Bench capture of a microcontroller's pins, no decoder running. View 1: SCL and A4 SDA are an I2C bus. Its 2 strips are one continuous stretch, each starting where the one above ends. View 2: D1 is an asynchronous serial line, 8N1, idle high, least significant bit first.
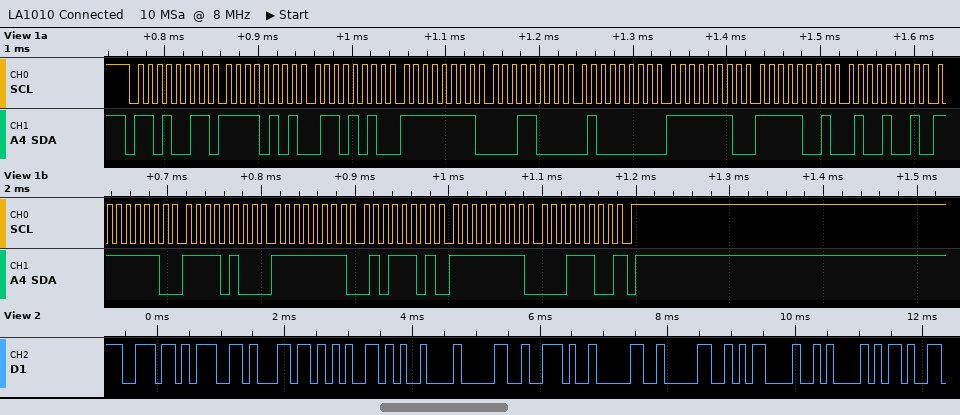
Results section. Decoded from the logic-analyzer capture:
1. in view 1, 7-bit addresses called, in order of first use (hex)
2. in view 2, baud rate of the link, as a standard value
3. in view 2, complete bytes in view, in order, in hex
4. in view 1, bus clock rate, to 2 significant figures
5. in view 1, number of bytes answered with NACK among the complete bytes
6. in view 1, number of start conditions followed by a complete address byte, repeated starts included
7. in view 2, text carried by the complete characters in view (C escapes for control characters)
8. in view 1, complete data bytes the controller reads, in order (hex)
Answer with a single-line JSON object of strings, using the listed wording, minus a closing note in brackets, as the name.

{"in view 1, 7-bit addresses called, in order of first use": "0x69", "in view 2, baud rate of the link, as a standard value": "9600 baud", "in view 2, complete bytes in view, in order, in hex": "6E 67 6C 65 09 30 2E 30 30 0D 0A 2D", "in view 1, bus clock rate, to 2 significant figures": "100 kHz", "in view 1, number of bytes answered with NACK among the complete bytes": "1", "in view 1, number of start conditions followed by a complete address byte, repeated starts included": "1", "in view 2, text carried by the complete characters in view": "\"ngle\\t0.00\\r\\n-\"", "in view 1, complete data bytes the controller reads, in order": "F5 6A FF 18 40 FE F9 49 FE F4 FF 5D FF 1C"}
